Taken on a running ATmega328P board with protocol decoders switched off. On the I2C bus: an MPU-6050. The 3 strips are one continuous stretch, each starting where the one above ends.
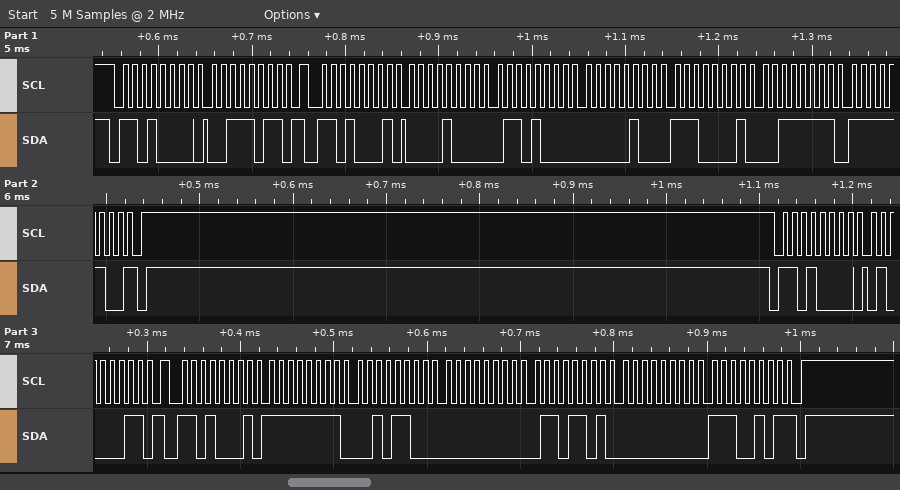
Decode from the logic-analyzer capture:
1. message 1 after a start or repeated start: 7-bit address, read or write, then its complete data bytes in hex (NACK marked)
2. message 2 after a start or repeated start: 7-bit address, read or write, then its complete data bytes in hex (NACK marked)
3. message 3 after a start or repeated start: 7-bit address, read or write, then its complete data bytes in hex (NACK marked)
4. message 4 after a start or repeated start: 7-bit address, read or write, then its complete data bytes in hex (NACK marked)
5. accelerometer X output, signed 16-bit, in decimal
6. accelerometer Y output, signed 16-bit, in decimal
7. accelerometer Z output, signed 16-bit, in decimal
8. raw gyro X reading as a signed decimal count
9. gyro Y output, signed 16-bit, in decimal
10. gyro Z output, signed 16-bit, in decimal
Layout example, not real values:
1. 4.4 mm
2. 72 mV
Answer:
1. 0x68 write: 3B
2. 0x68 read: 08 68 04 E1 3F FC NACK
3. 0x68 write: 43
4. 0x68 read: FF 2C 00 6D 00 E5 NACK
5. 2152
6. 1249
7. 16380
8. -212
9. 109
10. 229
